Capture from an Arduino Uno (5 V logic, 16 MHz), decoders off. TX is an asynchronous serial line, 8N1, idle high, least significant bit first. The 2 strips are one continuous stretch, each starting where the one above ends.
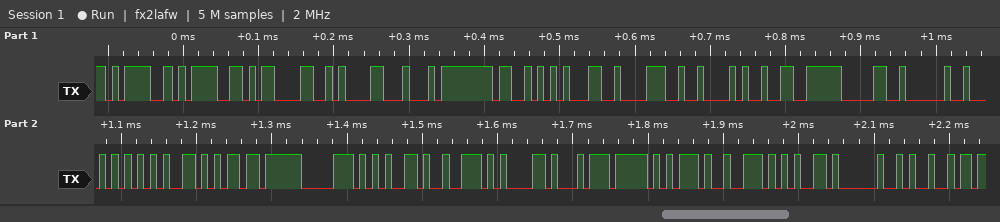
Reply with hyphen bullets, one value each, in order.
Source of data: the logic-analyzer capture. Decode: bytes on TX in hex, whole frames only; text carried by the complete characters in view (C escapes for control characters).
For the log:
- 0x3D 0x3D 0x0D 0x0A 0x44 0x53 0x31 0x38 0x42 0x32 0x30 0x20 0x54 0x65 0x6D 0x70 0x65 0x72 0x61 0x74 0x75 0x72 0x65 0x20 0x49
- "==\r\nDS18B20 Temperature I"
